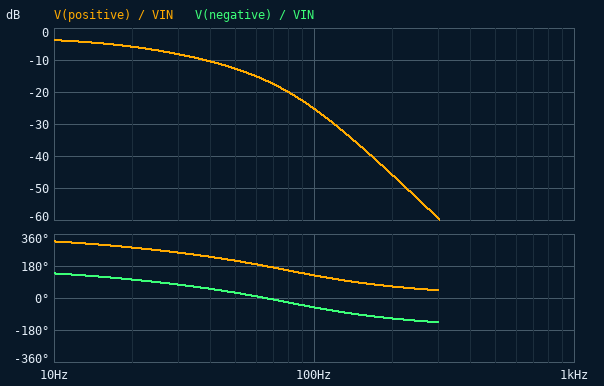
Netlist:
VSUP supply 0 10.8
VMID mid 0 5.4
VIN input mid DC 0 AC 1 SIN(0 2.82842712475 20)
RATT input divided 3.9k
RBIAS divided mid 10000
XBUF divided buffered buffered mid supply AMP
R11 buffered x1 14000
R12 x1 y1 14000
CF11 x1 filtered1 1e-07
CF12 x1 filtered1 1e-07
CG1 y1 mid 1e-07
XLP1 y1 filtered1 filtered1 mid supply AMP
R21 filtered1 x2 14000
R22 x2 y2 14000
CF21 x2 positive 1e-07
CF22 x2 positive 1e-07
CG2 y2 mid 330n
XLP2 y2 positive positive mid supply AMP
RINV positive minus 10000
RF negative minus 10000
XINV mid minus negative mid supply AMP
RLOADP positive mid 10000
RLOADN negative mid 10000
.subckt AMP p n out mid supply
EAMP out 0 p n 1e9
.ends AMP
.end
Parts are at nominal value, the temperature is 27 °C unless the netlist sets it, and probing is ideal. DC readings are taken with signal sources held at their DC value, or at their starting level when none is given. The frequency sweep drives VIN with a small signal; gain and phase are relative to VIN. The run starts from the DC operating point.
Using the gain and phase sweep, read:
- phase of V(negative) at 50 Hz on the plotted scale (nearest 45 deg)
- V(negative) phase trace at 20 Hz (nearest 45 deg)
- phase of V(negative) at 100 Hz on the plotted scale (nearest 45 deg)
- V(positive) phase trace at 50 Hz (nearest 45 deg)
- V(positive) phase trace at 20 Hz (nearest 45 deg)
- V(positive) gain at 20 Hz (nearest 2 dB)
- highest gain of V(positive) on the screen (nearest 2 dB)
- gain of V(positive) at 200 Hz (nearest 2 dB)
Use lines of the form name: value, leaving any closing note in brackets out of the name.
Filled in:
phase of V(negative) at 50 Hz on the plotted scale: 45 deg
V(negative) phase trace at 20 Hz: 90 deg
phase of V(negative) at 100 Hz on the plotted scale: -45 deg
V(positive) phase trace at 50 Hz: 225 deg
V(positive) phase trace at 20 Hz: 270 deg
V(positive) gain at 20 Hz: -6 dB
highest gain of V(positive) on the screen: -4 dB
gain of V(positive) at 200 Hz: -46 dB
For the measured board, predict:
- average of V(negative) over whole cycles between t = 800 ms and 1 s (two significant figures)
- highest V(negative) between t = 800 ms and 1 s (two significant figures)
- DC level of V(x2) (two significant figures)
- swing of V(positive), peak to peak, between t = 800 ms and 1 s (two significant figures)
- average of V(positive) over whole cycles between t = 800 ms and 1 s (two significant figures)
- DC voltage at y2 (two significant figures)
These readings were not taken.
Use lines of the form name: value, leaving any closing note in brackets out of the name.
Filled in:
average of V(negative) over whole cycles between t = 800 ms and 1 s: 5.4 V
highest V(negative) between t = 800 ms and 1 s: 6.8 V
DC level of V(x2): 5.4 V
swing of V(positive), peak to peak, between t = 800 ms and 1 s: 2.9 V
average of V(positive) over whole cycles between t = 800 ms and 1 s: 5.4 V
DC voltage at y2: 5.4 V
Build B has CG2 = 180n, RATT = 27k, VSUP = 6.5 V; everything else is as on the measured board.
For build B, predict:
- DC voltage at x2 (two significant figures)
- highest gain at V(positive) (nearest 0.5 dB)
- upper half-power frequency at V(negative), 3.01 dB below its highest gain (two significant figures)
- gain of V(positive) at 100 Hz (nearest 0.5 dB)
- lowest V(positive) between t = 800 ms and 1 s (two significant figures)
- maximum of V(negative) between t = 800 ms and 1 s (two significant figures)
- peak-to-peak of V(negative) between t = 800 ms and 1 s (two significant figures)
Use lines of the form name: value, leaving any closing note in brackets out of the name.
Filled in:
DC voltage at x2: 5.4 V
highest gain at V(positive): -11.5 dB
upper half-power frequency at V(negative), 3.01 dB below its highest gain: 40 Hz
gain of V(positive) at 100 Hz: -28.0 dB
lowest V(positive) between t = 800 ms and 1 s: 4.7 V
maximum of V(negative) between t = 800 ms and 1 s: 6.1 V
peak-to-peak of V(negative) between t = 800 ms and 1 s: 1.4 V
